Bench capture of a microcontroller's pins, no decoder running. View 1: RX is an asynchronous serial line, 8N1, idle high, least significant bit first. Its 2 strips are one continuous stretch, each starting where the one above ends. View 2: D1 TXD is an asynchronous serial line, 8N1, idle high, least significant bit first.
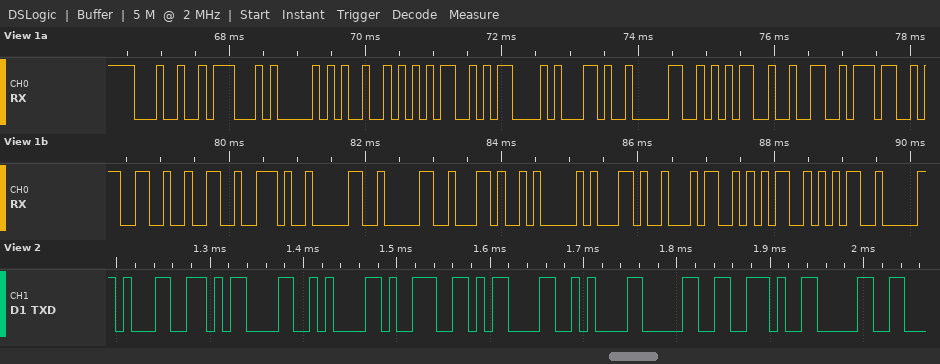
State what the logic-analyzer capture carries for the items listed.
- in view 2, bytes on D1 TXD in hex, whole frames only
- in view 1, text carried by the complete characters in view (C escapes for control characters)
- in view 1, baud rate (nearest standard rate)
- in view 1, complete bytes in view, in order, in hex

31 0D 0A 39 0D 0A 30 2E 30
"$GPRMC,052732.00,A,455"
9600 baud
0x24 0x47 0x50 0x52 0x4D 0x43 0x2C 0x30 0x35 0x32 0x37 0x33 0x32 0x2E 0x30 0x30 0x2C 0x41 0x2C 0x34 0x35 0x35
